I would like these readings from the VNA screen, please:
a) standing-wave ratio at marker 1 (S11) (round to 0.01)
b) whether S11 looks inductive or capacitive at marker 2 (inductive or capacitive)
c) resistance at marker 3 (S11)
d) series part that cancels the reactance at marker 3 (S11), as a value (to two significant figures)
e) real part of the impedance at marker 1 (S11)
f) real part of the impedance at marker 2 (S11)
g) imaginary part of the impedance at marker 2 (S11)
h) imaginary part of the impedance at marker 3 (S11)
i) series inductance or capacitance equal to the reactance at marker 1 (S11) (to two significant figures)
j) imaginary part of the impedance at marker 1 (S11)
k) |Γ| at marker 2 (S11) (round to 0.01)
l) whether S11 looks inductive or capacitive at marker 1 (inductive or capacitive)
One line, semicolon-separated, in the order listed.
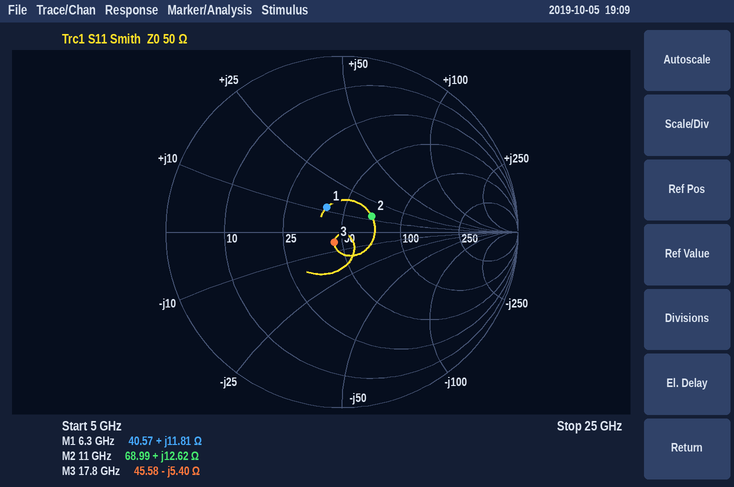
1.40; inductive; 45.58 Ω; 48 pH; 40.57 Ω; 68.99 Ω; +12.62 Ω; -5.40 Ω; 300 pH; +11.81 Ω; 0.19; inductive
